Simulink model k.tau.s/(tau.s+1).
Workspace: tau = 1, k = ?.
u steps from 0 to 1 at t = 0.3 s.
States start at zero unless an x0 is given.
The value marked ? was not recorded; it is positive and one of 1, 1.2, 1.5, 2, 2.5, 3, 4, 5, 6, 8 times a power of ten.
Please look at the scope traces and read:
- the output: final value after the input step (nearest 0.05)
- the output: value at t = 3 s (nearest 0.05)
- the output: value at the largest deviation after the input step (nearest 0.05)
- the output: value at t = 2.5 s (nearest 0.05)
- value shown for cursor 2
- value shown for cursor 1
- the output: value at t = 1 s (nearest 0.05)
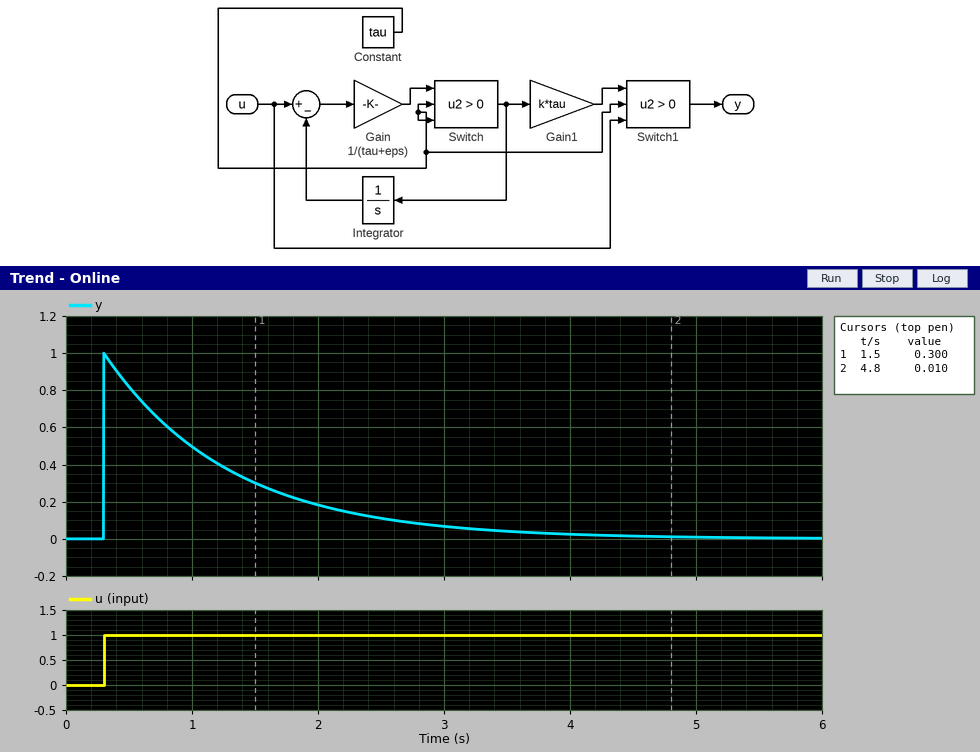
0.00
0.05
1.00
0.10
0.010
0.300
0.50
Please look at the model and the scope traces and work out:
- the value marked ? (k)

1
